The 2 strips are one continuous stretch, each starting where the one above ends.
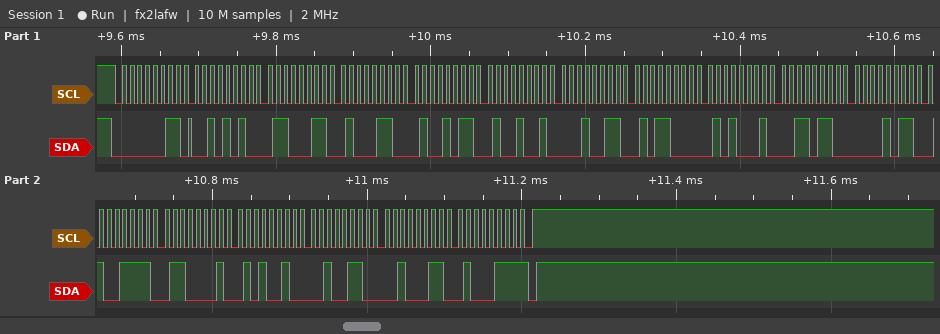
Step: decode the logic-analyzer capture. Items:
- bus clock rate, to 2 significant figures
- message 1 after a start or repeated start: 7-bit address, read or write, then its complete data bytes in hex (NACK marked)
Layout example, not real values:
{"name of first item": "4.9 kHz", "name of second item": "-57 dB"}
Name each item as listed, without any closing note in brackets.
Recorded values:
{"bus clock rate, to 2 significant figures": "100 kHz", "message 1 after a start or repeated start: 7-bit address, read or write, then its complete data bytes in hex": "0x01 read: 2A 63 46 4B 49 13 58 51 36 0B 4F 61 52 26 23 47 NACK"}
